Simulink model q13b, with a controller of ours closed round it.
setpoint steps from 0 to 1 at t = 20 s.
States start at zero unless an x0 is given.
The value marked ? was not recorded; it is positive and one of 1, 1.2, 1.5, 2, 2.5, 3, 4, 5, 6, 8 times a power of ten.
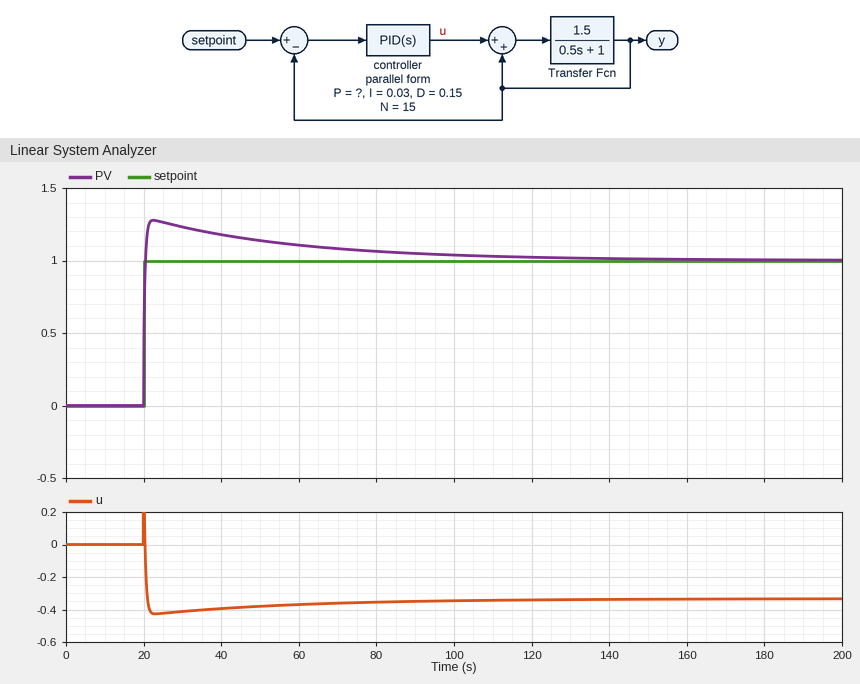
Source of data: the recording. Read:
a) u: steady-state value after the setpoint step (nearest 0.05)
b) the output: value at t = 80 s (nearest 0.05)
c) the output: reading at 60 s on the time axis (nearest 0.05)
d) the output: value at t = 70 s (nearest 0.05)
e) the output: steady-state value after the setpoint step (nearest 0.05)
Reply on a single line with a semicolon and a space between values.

-0.35; 1.05; 1.10; 1.10; 1.00
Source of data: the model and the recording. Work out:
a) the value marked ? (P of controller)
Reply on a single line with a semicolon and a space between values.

1.5
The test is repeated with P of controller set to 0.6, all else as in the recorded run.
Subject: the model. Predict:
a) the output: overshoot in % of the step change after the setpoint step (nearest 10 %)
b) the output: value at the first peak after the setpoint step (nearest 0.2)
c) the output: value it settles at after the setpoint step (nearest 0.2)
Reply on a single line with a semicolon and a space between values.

100 %; 2.0; 1.0
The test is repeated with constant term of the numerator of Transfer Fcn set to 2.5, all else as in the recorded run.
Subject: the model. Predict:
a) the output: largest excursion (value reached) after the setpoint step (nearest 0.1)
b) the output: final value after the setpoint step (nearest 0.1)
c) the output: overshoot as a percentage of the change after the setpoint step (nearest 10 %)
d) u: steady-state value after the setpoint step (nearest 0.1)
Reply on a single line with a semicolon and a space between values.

1.6; 1.0; 60 %; -0.6
